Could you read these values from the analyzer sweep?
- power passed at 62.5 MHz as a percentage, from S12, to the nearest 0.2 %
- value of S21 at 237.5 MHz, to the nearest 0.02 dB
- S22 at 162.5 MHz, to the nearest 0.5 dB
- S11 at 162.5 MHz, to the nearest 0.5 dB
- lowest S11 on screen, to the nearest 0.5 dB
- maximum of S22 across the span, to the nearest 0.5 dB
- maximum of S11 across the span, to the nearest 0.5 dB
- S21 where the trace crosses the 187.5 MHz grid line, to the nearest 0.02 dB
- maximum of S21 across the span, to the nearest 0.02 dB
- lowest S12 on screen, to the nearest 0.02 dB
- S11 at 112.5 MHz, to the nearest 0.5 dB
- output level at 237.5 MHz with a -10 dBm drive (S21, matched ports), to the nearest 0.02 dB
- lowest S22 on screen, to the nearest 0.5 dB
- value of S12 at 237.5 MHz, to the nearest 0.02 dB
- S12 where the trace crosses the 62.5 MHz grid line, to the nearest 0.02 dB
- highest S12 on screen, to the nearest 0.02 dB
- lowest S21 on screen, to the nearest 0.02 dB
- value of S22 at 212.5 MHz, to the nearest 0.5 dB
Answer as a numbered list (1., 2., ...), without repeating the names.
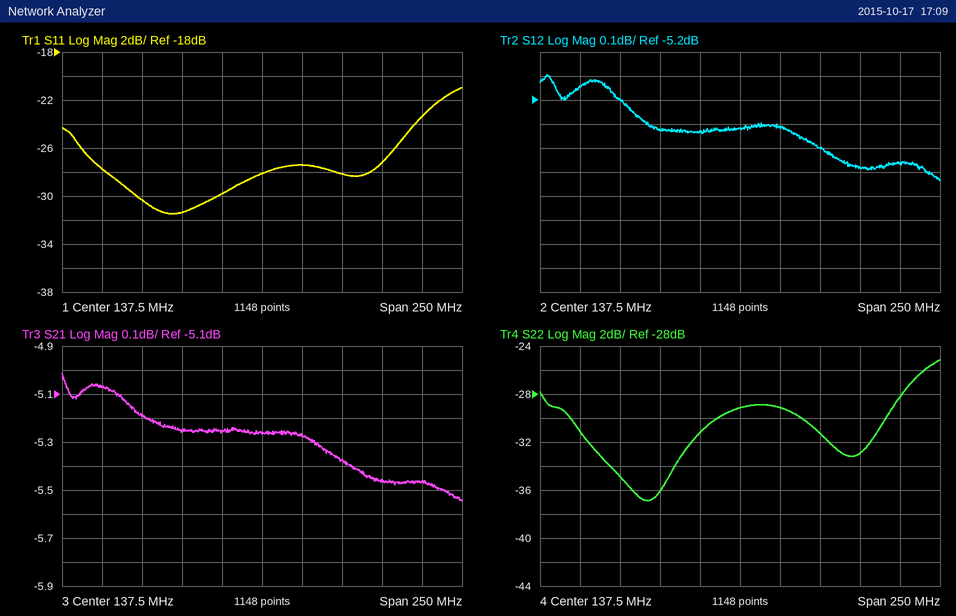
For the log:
1. 30.2 %
2. -5.46 dB
3. -29.0 dB
4. -27.5 dB
5. -31.5 dB
6. -25.0 dB
7. -21.0 dB
8. -5.38 dB
9. -5.02 dB
10. -5.54 dB
11. -30.0 dB
12. -15.46 dBm
13. -37.0 dB
14. -5.46 dB
15. -5.20 dB
16. -5.10 dB
17. -5.54 dB
18. -33.0 dB
